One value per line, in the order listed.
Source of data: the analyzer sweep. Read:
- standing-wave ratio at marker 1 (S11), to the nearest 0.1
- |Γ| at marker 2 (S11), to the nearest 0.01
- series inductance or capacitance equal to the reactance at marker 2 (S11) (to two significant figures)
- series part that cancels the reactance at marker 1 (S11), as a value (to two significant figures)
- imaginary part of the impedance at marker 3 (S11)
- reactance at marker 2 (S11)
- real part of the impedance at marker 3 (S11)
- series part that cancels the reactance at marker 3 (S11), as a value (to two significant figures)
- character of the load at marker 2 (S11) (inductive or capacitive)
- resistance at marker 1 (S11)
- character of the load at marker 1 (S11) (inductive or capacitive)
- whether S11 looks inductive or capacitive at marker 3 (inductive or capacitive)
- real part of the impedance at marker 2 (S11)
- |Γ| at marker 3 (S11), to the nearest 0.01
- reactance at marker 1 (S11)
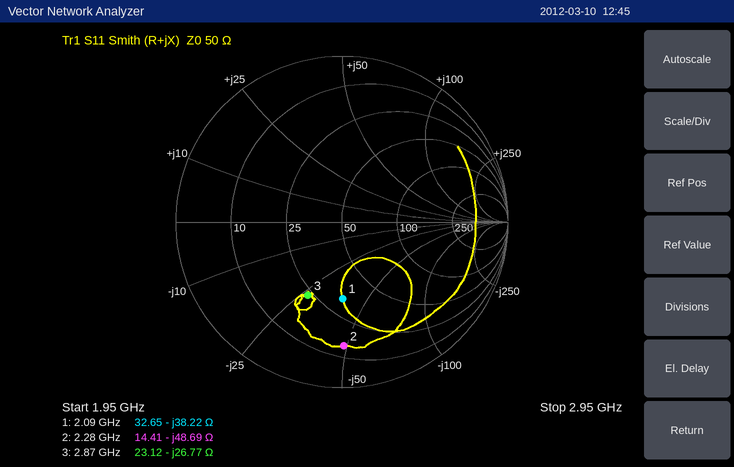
2.7
0.75
1.4 pF
2.9 nH
-26.77 Ω
-48.69 Ω
23.12 Ω
1.5 nH
capacitive
32.65 Ω
capacitive
capacitive
14.41 Ω
0.49
-38.22 Ω
